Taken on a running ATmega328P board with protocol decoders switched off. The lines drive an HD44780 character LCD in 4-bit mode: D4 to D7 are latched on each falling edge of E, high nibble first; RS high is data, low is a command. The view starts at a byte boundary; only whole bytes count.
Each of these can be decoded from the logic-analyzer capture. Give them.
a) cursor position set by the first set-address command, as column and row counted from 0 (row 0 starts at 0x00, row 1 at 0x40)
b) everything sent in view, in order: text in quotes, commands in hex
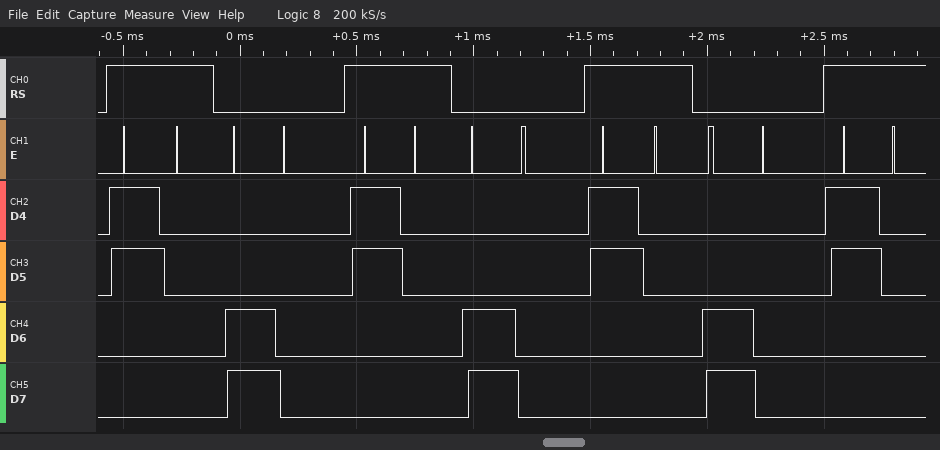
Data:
column 0, row 1
"0" 0xC0 "0" 0xC0 "0" 0xC0 "0"
